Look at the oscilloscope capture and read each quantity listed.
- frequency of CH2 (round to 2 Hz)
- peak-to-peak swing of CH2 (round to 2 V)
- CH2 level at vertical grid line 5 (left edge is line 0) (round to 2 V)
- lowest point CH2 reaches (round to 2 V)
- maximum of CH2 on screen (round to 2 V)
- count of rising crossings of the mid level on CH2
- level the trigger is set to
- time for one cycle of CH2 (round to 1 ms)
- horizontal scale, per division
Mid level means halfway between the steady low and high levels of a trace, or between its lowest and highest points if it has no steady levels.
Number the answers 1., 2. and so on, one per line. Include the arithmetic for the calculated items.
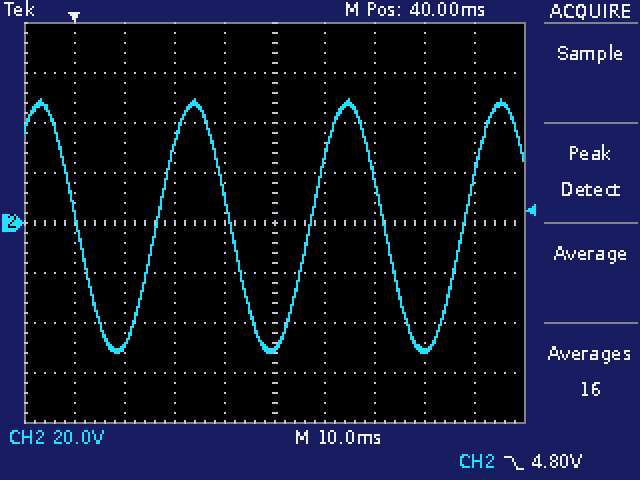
1. 1 / 31 ms ≈ 32 Hz
2. 50 V − (-52 V) = 102 V
3. -50 V
4. -52 V
5. 50 V
6. 3
7. 4.80 V
8. 31 ms
9. 10 ms
